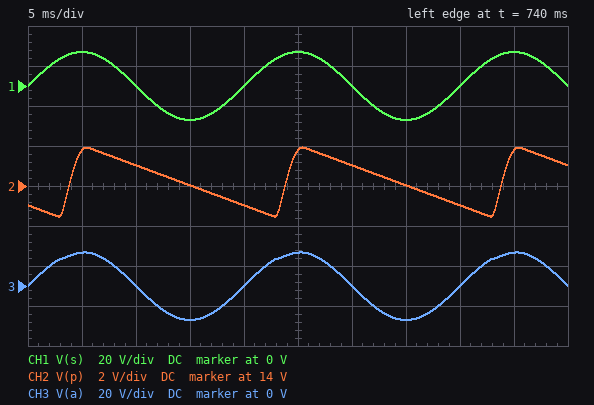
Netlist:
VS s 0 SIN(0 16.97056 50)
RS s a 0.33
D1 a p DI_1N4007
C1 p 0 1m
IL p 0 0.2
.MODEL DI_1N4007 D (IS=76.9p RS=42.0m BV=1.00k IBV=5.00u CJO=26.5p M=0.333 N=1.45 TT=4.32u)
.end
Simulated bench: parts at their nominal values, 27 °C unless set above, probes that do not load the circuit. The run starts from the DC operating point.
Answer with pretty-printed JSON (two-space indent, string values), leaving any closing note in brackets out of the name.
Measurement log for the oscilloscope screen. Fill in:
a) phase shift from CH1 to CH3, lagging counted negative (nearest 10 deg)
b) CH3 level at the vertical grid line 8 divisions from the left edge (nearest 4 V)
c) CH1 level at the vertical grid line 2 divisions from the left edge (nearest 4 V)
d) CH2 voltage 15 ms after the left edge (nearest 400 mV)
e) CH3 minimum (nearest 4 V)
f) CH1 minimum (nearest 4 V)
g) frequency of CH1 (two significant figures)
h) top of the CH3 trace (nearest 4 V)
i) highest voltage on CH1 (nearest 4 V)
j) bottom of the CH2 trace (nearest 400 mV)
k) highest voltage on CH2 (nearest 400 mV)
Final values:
{
  "phase shift from CH1 to CH3, lagging counted negative": "0 deg",
  "CH3 level at the vertical grid line 8 divisions from the left edge": "0 V",
  "CH1 level at the vertical grid line 2 divisions from the left edge": "0 V",
  "CH2 voltage 15 ms after the left edge": "14.0 V",
  "CH3 minimum": "-16 V",
  "CH1 minimum": "-16 V",
  "frequency of CH1": "50 Hz",
  "top of the CH3 trace": "16 V",
  "highest voltage on CH1": "16 V",
  "bottom of the CH2 trace": "12.4 V",
  "highest voltage on CH2": "16.0 V"
}
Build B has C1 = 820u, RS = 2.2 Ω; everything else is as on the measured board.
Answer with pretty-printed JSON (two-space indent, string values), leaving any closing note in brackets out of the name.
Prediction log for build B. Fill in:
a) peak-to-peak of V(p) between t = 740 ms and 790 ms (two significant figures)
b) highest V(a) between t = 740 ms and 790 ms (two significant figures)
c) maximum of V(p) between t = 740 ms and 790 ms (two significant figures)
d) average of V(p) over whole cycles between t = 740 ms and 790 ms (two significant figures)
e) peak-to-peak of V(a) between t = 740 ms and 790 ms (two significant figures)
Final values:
{
  "peak-to-peak of V(p) between t = 740 ms and 790 ms": "3.9 V",
  "highest V(a) between t = 740 ms and 790 ms": "15 V",
  "maximum of V(p) between t = 740 ms and 790 ms": "14 V",
  "average of V(p) over whole cycles between t = 740 ms and 790 ms": "12 V",
  "peak-to-peak of V(a) between t = 740 ms and 790 ms": "32 V"
}
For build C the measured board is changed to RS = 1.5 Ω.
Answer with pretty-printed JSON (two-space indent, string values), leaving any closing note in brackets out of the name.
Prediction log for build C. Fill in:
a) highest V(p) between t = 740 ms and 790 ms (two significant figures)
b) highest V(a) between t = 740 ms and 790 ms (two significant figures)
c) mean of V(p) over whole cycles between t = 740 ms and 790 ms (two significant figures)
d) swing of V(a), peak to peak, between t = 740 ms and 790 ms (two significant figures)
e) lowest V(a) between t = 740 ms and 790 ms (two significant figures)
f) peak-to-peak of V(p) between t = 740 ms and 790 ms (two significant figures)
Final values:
{
  "highest V(p) between t = 740 ms and 790 ms": "15 V",
  "highest V(a) between t = 740 ms and 790 ms": "16 V",
  "mean of V(p) over whole cycles between t = 740 ms and 790 ms": "13 V",
  "swing of V(a), peak to peak, between t = 740 ms and 790 ms": "33 V",
  "lowest V(a) between t = 740 ms and 790 ms": "-17 V",
  "peak-to-peak of V(p) between t = 740 ms and 790 ms": "3.3 V"
}
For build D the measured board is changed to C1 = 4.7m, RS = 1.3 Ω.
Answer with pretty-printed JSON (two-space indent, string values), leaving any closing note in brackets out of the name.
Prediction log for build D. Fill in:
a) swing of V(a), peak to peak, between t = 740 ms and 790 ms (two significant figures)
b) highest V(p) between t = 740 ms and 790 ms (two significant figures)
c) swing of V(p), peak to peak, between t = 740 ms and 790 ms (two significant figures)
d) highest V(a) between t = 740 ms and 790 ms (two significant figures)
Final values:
{
  "swing of V(a), peak to peak, between t = 740 ms and 790 ms": "32 V",
  "highest V(p) between t = 740 ms and 790 ms": "14 V",
  "swing of V(p), peak to peak, between t = 740 ms and 790 ms": "710 mV",
  "highest V(a) between t = 740 ms and 790 ms": "15 V"
}
